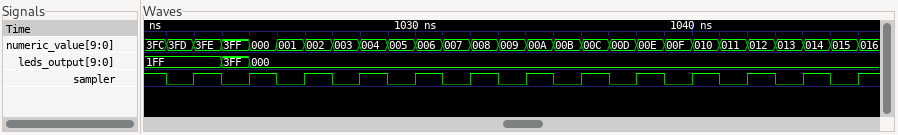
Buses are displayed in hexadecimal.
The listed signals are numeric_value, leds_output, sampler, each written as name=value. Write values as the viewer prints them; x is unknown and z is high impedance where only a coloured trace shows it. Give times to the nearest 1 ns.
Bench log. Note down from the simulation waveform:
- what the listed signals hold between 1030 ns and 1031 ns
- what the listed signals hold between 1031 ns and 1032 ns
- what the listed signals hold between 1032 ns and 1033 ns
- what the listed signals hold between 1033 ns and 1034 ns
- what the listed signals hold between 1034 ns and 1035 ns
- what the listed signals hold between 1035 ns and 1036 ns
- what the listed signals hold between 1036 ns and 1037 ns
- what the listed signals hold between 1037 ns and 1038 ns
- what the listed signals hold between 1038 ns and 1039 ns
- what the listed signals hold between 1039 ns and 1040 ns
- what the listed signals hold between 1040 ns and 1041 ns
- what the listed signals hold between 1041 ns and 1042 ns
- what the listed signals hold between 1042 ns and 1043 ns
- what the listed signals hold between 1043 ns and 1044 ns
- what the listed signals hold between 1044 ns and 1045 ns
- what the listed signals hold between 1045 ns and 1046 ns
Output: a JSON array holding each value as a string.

["numeric_value=006, leds_output=000, sampler=1", "numeric_value=007, leds_output=000, sampler=0", "numeric_value=008, leds_output=000, sampler=1", "numeric_value=009, leds_output=000, sampler=0", "numeric_value=00A, leds_output=000, sampler=1", "numeric_value=00B, leds_output=000, sampler=0", "numeric_value=00C, leds_output=000, sampler=1", "numeric_value=00D, leds_output=000, sampler=0", "numeric_value=00E, leds_output=000, sampler=1", "numeric_value=00F, leds_output=000, sampler=0", "numeric_value=010, leds_output=000, sampler=1", "numeric_value=011, leds_output=000, sampler=0", "numeric_value=012, leds_output=000, sampler=1", "numeric_value=013, leds_output=000, sampler=0", "numeric_value=014, leds_output=000, sampler=1", "numeric_value=015, leds_output=000, sampler=0"]
